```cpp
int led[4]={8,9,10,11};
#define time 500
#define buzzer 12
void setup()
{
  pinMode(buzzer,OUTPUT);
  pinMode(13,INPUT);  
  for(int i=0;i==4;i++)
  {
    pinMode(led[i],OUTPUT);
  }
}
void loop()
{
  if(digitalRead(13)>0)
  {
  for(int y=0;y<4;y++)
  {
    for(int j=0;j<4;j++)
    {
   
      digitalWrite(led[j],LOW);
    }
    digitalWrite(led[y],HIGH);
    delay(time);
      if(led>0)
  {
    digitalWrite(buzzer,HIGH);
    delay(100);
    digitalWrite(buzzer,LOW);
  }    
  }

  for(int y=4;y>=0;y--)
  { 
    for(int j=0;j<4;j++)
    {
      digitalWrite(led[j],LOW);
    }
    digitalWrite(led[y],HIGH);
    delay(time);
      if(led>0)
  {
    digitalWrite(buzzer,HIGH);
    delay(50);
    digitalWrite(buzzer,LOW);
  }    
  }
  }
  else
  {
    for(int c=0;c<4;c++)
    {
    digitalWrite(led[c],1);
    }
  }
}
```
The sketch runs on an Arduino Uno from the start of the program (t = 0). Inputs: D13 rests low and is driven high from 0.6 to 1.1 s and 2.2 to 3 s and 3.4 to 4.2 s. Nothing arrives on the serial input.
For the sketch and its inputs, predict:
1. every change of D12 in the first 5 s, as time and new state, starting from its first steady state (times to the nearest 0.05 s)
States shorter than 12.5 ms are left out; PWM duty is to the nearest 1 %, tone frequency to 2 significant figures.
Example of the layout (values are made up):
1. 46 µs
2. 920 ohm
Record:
1. 0 s low; 1.1 s high; 1.2 s low; 1.7 s high; 1.8 s low; 2.3 s high; 2.4 s low; 2.9 s high; 3 s low; 3.5 s high; 3.55 s low; 4.05 s high; 4.1 s low; 4.6 s high; 4.65 s low
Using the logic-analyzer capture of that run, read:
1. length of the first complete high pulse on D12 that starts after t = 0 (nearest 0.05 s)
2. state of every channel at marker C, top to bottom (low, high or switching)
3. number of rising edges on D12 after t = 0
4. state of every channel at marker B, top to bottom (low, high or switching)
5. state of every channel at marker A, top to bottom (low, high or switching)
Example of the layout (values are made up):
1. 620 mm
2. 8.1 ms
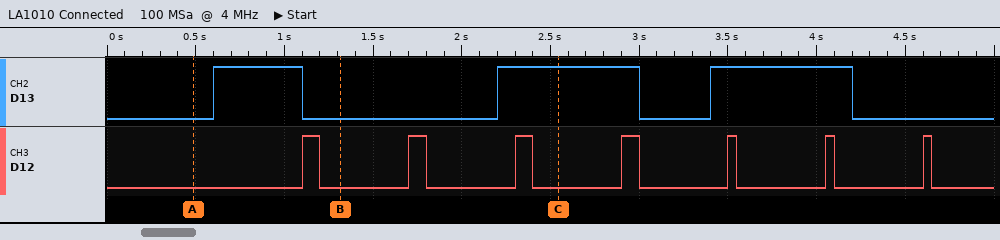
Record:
1. 0.10 s
2. D13 high, D12 low
3. 7
4. D13 low, D12 low
5. D13 low, D12 low
